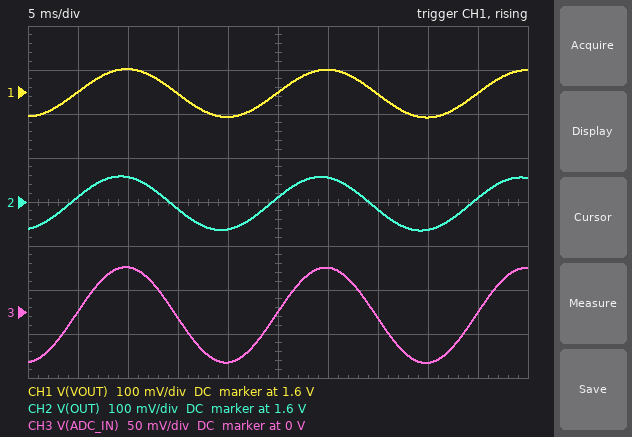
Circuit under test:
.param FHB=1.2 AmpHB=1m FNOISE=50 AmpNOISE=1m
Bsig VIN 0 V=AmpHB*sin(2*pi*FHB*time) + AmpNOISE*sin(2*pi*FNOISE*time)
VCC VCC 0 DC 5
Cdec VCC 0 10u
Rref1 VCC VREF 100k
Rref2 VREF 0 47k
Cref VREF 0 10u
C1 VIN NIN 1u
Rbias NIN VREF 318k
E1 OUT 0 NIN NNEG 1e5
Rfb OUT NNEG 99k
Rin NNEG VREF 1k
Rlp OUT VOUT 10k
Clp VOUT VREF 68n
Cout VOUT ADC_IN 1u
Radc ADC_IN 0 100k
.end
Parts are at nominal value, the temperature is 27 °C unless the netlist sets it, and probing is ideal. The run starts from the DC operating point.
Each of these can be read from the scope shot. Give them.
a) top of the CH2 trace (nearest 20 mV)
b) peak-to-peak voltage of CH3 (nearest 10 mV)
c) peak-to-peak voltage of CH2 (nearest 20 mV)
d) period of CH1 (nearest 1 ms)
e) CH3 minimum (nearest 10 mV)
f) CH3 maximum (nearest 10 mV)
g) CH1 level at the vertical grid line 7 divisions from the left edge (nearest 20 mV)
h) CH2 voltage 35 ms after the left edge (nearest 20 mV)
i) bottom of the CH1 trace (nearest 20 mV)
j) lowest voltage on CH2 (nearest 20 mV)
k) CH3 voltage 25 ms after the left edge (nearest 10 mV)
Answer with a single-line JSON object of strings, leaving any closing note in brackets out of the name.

{"top of the CH2 trace": "1.66 V", "peak-to-peak voltage of CH3": "110 mV", "peak-to-peak voltage of CH2": "120 mV", "period of CH1": "20 ms", "CH3 minimum": "-60 mV", "CH3 maximum": "50 mV", "CH1 level at the vertical grid line 7 divisions from the left edge": "1.60 V", "CH2 voltage 35 ms after the left edge": "1.58 V", "bottom of the CH1 trace": "1.54 V", "lowest voltage on CH2": "1.54 V", "CH3 voltage 25 ms after the left edge": "0 V"}
